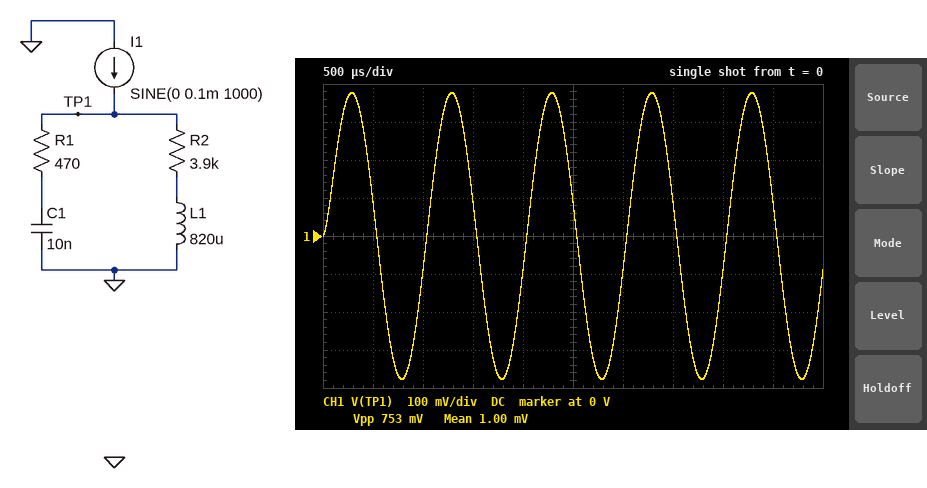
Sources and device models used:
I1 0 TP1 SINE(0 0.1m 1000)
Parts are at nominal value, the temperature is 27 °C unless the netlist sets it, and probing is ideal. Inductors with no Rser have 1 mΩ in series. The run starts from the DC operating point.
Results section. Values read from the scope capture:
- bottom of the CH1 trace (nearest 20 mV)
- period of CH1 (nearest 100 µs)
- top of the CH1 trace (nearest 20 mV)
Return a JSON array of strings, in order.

["-380 mV", "1.0 ms", "380 mV"]
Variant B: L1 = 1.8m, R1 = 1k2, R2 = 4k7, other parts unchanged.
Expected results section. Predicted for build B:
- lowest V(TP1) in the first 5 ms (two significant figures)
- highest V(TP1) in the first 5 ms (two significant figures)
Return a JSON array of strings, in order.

["-440 mV", "440 mV"]
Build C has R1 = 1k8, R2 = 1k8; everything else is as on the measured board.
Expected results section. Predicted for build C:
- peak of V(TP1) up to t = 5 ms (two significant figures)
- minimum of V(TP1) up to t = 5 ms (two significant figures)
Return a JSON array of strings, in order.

["180 mV", "-180 mV"]
